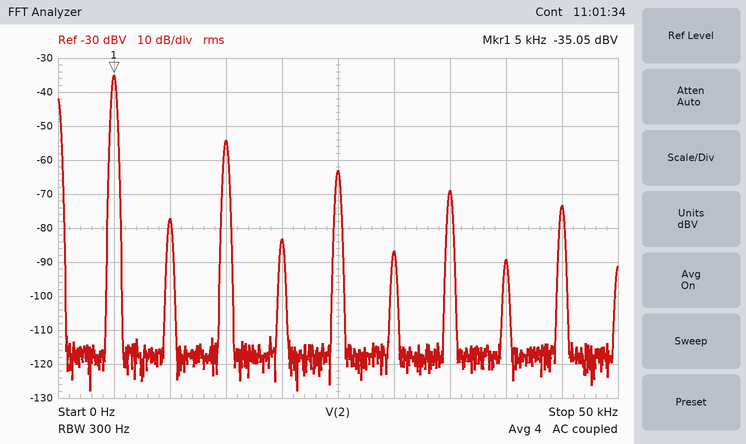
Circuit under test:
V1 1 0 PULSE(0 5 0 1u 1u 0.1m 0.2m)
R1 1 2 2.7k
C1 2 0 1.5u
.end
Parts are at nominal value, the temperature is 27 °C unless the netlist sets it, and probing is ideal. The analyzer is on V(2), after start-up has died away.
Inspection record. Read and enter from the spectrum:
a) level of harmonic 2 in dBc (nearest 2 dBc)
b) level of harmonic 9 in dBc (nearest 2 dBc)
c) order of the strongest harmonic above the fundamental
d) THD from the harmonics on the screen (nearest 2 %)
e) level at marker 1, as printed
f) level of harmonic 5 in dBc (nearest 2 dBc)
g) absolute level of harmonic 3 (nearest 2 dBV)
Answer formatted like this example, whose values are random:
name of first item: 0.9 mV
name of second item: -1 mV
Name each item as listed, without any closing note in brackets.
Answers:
level of harmonic 2 in dBc: -42 dBc
level of harmonic 9 in dBc: -38 dBc
order of the strongest harmonic above the fundamental: 3
THD from the harmonics on the screen: 12 %
level at marker 1, as printed: -35.05 dBV
level of harmonic 5 in dBc: -28 dBc
absolute level of harmonic 3: -54 dBV
